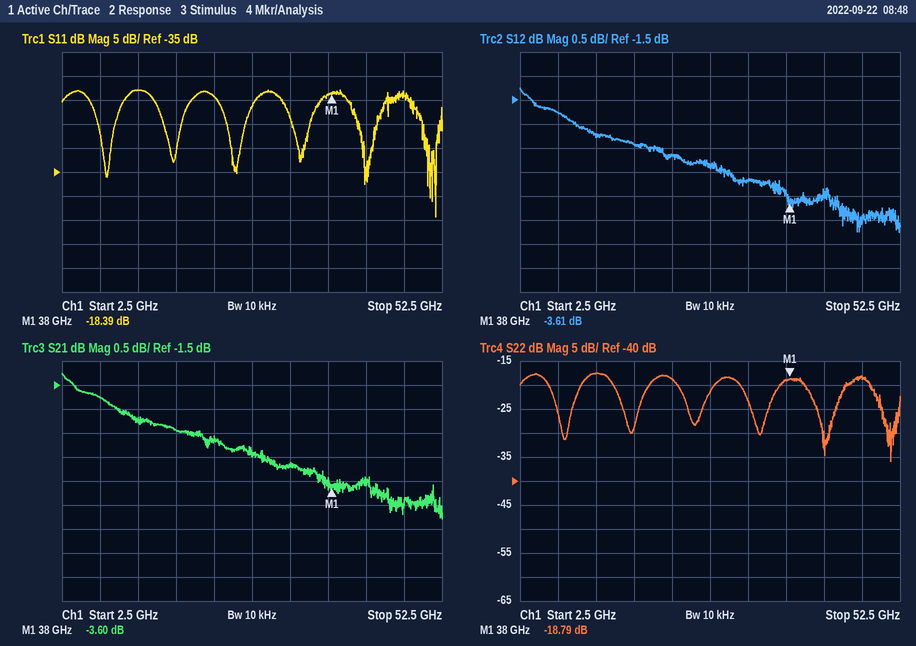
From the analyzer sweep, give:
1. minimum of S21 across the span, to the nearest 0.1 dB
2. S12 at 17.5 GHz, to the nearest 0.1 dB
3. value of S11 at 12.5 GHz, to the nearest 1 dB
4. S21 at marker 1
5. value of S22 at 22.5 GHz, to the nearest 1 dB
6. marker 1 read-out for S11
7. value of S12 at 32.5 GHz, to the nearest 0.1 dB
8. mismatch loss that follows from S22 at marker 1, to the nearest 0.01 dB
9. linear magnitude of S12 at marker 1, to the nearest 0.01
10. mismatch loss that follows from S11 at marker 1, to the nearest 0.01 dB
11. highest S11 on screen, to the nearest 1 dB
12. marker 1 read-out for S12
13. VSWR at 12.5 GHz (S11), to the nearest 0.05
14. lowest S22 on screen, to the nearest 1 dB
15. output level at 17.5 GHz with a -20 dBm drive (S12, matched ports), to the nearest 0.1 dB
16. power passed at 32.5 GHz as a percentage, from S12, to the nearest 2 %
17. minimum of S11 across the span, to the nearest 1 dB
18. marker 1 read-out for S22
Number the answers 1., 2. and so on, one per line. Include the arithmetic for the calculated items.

1. -4.3 dB
2. -2.4 dB
3. -18 dB
4. -3.60 dB
5. -19 dB
6. -18.39 dB
7. -3.2 dB
8. −10 log10(1 − 10^(-18.79/10)) ≈ 0.06 dB
9. 10^(-3.61/20) ≈ 0.66
10. −10 log10(1 − 10^(-18.39/10)) ≈ 0.06 dB
11. -18 dB
12. -3.61 dB
13. |Γ| = 10^(-18/20) = 0.1259; VSWR = (1 + 0.1259)/(1 − 0.1259) ≈ 1.29, so 1.30 to the nearest 0.05
14. -36 dB
15. -20 dBm + (-2.4 dB) = -22.4 dBm
16. 10^(-3.2/10) ≈ 48 %
17. -44 dB
18. -18.79 dB
